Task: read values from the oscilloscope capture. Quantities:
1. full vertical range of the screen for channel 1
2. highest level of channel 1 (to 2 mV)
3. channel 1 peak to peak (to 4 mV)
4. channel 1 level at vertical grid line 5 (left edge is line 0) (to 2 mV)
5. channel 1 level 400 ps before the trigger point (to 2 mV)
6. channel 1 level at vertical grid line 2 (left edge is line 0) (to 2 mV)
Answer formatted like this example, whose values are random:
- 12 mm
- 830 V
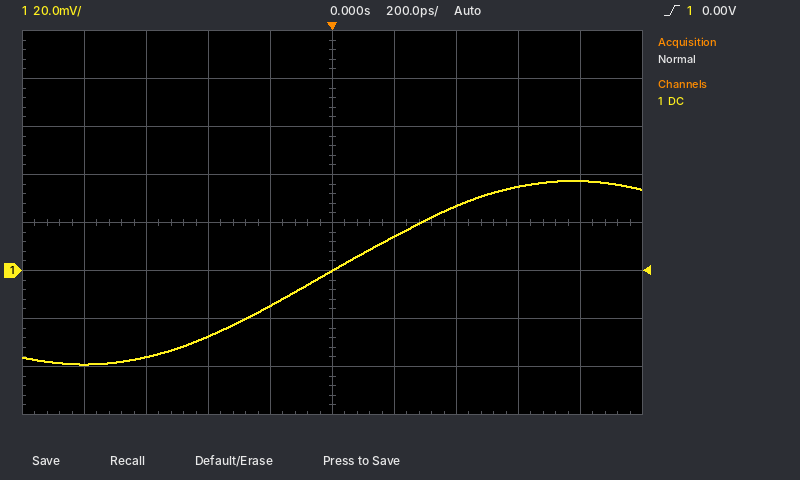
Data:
- 160 mV
- 38 mV
- 76 mV
- 0 mV
- -28 mV
- -36 mV
